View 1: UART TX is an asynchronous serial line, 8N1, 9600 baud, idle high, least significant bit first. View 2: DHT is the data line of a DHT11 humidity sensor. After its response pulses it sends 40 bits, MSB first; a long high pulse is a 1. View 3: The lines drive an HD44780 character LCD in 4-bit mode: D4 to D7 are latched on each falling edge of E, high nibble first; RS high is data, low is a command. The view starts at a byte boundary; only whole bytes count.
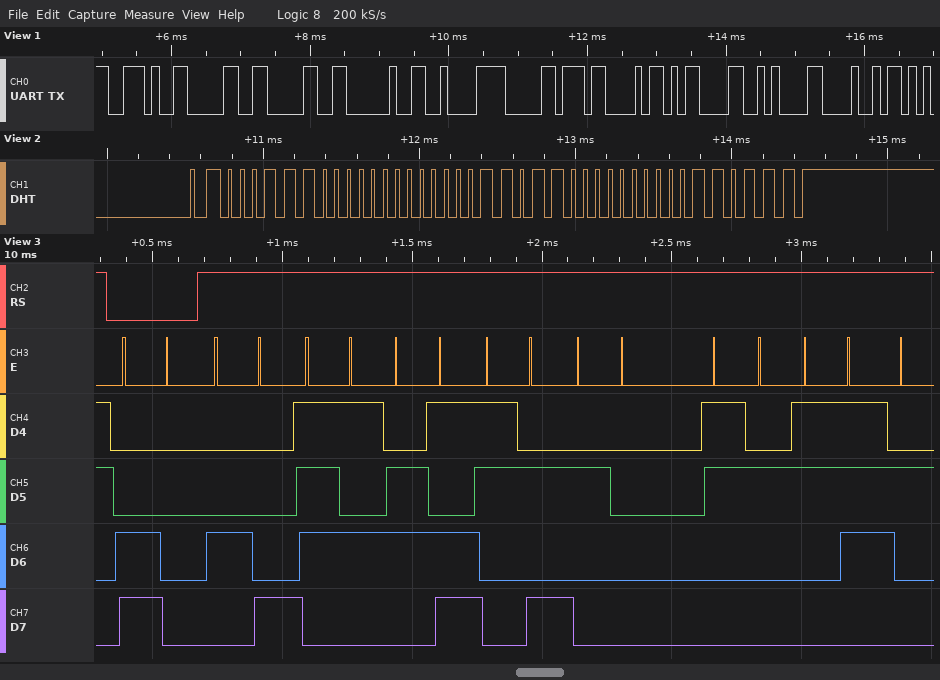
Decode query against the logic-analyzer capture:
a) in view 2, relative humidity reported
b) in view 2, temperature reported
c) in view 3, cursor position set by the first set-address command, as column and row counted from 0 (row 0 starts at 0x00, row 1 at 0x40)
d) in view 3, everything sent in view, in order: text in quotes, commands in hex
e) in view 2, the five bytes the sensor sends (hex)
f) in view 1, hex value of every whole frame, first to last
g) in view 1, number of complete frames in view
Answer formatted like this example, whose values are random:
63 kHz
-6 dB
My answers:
28 %
27.0 °C
column 0, row 1
0xC0 "Hum: 27"
1C 00 1B 00 37
2E 30 30 20 C2 B0 43 0D 0A 48
10
